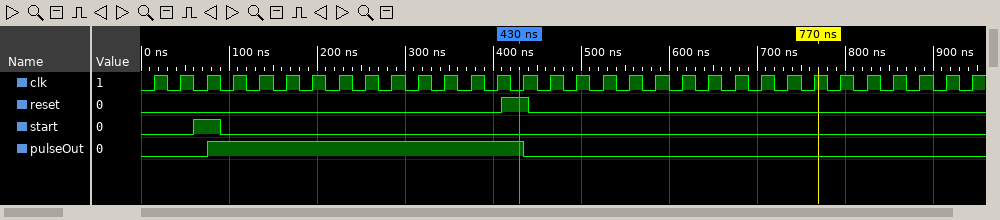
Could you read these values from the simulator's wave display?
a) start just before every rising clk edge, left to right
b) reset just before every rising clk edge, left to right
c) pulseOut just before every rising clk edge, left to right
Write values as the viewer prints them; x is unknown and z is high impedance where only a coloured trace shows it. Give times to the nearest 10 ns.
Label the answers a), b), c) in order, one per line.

a) 0 0 1 0 0 0 0 0 0 0 0 0 0 0 0 0 0 0 0 0 0 0 0 0 0 0 0 0 0 0 0 0
b) 0 0 0 0 0 0 0 0 0 0 0 0 0 0 1 0 0 0 0 0 0 0 0 0 0 0 0 0 0 0 0 0
c) 0 0 0 1 1 1 1 1 1 1 1 1 1 1 1 0 0 0 0 0 0 0 0 0 0 0 0 0 0 0 0 0
